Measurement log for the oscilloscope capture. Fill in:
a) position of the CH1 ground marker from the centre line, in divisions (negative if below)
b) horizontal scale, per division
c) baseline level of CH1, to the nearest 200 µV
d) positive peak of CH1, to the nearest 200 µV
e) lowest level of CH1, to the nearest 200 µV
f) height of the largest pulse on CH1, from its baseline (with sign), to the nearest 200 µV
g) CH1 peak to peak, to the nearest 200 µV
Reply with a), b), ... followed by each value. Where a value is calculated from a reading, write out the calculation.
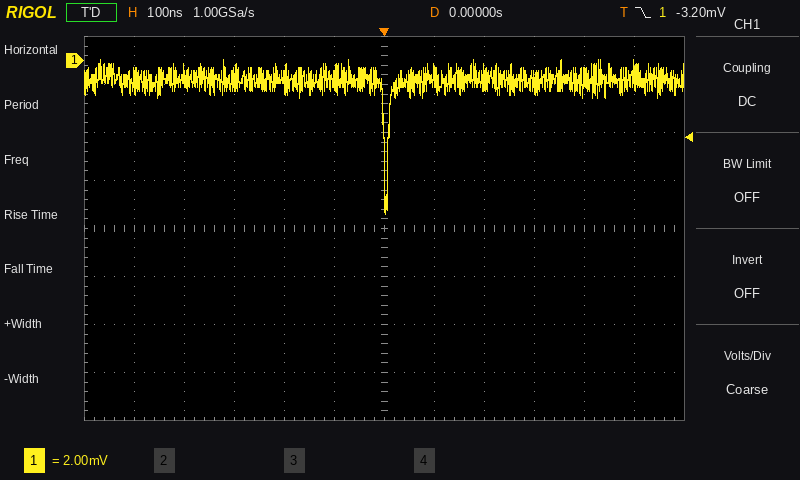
a) +3.5 div
b) 100 ns
c) -800 µV
d) 0.0 mV
e) -6.4 mV
f) -6.4 mV − (-800 µV) = -5.6 mV
g) 0.0 mV − (-6.4 mV) = 6.4 mV
